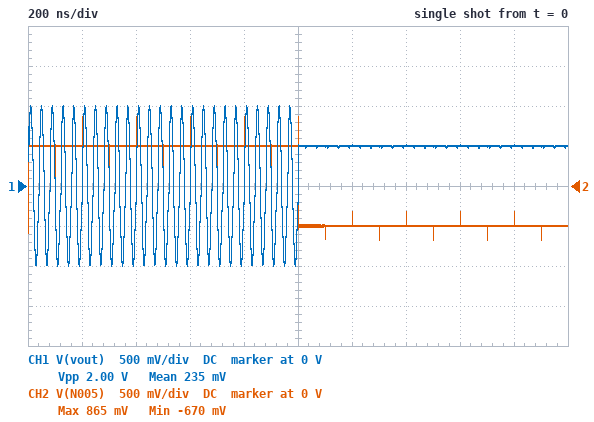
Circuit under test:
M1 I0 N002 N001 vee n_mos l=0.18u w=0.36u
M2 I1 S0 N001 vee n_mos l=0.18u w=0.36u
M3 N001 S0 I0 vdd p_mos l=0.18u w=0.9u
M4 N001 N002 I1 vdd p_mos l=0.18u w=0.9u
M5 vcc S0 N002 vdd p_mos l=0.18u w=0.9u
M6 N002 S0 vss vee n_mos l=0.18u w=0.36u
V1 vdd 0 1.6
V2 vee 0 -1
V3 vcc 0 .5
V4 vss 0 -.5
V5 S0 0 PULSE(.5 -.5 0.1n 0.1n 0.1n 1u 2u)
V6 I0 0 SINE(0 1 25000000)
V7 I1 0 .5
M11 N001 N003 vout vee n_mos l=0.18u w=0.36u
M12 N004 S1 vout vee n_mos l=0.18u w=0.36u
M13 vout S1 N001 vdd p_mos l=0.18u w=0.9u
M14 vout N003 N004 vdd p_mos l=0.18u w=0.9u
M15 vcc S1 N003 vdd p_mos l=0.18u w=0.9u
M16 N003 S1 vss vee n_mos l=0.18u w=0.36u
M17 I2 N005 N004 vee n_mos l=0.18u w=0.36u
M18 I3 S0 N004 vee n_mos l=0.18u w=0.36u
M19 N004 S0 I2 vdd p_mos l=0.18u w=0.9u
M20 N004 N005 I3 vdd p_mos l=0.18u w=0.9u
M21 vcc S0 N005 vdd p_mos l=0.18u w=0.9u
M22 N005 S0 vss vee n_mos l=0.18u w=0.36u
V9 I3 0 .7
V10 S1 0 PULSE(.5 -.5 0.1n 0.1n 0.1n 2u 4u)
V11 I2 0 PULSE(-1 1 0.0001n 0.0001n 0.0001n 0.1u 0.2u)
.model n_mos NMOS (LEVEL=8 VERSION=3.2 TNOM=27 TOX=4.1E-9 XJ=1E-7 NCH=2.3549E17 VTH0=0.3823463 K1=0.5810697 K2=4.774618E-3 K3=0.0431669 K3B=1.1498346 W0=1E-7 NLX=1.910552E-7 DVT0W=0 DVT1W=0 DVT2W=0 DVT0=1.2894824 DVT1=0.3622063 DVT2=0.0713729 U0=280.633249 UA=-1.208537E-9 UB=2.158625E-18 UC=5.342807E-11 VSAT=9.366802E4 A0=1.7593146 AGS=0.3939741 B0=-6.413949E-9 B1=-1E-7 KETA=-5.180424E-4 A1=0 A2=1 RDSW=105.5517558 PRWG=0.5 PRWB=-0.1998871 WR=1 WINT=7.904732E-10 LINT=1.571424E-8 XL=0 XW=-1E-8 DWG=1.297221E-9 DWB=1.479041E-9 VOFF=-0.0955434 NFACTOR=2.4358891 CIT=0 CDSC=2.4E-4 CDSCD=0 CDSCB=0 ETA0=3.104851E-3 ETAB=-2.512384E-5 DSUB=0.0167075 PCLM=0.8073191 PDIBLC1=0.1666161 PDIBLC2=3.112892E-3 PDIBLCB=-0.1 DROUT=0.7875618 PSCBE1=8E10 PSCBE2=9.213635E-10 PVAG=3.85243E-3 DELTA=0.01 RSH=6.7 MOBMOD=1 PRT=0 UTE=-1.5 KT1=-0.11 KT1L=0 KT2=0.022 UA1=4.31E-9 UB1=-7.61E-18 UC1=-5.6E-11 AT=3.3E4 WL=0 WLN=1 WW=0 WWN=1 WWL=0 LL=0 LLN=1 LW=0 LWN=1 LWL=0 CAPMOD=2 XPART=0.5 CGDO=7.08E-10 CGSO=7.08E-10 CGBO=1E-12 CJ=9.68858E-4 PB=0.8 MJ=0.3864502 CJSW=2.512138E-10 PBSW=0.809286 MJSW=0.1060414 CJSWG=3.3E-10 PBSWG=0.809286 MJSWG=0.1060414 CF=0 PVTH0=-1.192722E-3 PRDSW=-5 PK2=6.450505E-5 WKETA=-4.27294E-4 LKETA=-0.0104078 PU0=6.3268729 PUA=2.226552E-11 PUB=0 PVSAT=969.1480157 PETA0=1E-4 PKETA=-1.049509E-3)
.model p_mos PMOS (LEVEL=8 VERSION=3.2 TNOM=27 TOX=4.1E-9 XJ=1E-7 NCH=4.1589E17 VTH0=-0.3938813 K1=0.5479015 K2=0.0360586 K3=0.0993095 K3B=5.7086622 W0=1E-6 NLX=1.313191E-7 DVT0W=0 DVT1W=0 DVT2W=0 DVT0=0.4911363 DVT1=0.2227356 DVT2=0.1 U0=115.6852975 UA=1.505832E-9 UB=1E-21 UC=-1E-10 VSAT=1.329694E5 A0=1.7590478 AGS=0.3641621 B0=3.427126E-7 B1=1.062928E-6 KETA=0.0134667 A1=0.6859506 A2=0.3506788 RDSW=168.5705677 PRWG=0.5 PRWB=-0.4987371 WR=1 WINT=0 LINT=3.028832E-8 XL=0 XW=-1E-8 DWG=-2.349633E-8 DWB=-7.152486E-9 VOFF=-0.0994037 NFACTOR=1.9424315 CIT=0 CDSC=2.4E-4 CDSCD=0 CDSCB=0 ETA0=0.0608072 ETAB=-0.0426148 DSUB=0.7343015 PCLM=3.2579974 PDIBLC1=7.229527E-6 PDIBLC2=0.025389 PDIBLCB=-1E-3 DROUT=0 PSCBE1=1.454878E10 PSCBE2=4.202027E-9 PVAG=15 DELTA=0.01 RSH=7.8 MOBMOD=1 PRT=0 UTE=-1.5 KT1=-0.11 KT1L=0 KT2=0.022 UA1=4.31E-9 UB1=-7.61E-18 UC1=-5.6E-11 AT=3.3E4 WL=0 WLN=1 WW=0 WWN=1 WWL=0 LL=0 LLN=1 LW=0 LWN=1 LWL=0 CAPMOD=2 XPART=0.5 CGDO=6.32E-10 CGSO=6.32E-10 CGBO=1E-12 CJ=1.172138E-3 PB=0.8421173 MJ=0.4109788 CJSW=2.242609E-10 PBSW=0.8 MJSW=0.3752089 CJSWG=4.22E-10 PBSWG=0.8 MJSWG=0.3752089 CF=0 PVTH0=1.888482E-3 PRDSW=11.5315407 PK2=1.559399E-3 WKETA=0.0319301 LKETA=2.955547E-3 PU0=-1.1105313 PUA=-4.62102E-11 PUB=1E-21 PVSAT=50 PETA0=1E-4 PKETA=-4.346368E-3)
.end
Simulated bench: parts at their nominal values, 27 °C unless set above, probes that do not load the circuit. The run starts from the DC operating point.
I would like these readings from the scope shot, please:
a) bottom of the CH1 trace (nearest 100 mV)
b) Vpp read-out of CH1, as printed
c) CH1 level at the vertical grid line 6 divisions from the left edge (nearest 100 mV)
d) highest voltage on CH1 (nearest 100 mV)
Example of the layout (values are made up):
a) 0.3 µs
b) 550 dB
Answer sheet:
a) -1.0 V
b) 2.00 V
c) 500 mV
d) 1.0 V
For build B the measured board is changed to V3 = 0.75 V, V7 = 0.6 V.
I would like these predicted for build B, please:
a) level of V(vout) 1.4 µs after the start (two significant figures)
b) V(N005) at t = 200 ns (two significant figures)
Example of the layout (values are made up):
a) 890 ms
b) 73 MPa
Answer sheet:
a) 600 mV
b) 750 mV
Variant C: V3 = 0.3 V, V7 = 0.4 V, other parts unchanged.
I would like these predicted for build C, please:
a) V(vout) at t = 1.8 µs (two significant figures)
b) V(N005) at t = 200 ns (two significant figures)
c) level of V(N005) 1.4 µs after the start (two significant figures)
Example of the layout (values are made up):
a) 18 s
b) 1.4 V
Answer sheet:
a) 400 mV
b) 300 mV
c) -500 mV
